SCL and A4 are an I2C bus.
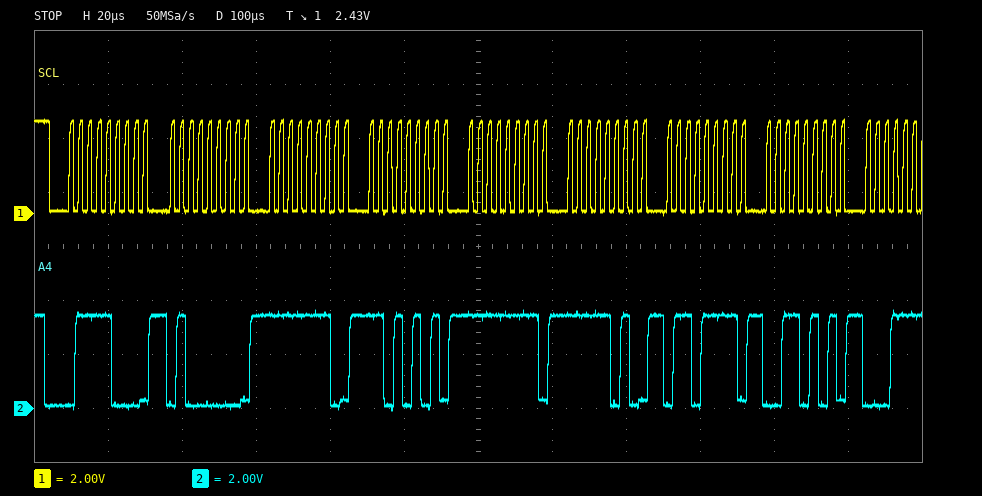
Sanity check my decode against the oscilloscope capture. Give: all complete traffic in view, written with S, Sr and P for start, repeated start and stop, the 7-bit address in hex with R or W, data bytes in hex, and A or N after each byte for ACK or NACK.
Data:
S 3CW A 40 A FE A D5 A FF A FA A 6F A 35 A
